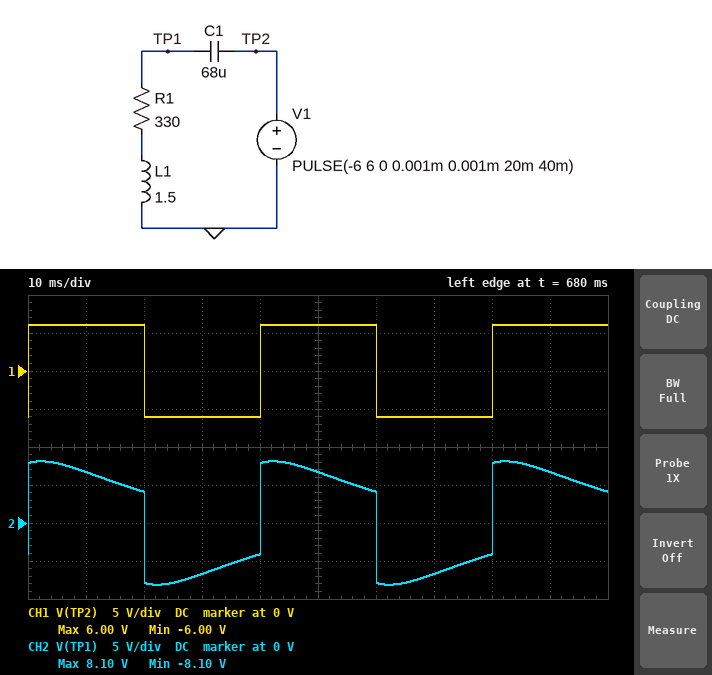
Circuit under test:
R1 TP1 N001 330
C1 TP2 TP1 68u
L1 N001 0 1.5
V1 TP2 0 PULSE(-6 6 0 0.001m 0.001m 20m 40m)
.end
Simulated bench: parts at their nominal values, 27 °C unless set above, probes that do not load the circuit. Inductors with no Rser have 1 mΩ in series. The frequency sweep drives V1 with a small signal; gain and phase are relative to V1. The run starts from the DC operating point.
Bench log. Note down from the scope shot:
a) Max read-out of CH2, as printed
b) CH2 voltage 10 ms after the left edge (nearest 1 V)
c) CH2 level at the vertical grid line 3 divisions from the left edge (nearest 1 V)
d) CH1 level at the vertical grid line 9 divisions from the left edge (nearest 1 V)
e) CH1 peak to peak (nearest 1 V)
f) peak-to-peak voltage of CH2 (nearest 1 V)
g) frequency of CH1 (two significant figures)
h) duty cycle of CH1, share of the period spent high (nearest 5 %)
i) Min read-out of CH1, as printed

8.10 V
7 V
-7 V
6 V
12 V
16 V
25 Hz
50 %
-6.00 V
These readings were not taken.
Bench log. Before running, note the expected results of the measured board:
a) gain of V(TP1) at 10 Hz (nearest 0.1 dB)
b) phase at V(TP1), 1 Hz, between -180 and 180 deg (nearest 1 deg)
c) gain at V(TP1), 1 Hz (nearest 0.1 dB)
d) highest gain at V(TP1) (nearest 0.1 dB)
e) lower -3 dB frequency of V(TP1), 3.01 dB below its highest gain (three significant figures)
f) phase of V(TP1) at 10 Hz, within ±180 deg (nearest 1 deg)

-0.4 dB
84 deg
-17.1 dB
1.1 dB
7.11 Hz
39 deg
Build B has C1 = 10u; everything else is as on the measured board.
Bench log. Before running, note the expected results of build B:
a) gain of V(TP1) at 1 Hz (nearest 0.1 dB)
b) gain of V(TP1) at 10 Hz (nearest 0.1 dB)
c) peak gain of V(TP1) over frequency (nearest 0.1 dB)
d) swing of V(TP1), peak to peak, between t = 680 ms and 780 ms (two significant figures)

-33.7 dB
-13.0 dB
4.1 dB
25 V
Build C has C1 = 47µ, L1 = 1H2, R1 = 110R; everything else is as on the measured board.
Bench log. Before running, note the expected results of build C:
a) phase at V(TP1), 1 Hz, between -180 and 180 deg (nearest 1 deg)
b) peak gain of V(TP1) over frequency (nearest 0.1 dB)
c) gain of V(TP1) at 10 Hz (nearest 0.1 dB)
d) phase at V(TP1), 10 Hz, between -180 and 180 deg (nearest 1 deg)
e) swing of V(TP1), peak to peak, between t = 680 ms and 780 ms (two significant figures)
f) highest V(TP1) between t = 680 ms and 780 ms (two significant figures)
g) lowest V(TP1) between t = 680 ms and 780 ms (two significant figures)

92 deg
5.2 dB
-6.6 dB
102 deg
29 V
15 V
-15 V
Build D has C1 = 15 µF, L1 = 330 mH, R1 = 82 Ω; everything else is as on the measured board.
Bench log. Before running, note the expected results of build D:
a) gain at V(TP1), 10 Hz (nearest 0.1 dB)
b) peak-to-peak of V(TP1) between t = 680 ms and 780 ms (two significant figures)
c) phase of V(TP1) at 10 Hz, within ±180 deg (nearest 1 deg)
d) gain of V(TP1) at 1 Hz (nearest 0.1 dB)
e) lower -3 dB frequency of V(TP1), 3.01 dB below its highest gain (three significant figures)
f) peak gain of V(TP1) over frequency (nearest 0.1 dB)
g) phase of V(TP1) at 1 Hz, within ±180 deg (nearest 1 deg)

-21.8 dB
25 V
100 deg
-42.2 dB
59.4 Hz
6.5 dB
91 deg
